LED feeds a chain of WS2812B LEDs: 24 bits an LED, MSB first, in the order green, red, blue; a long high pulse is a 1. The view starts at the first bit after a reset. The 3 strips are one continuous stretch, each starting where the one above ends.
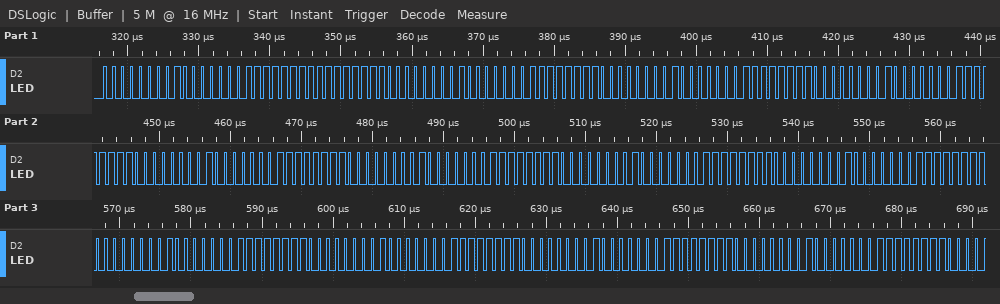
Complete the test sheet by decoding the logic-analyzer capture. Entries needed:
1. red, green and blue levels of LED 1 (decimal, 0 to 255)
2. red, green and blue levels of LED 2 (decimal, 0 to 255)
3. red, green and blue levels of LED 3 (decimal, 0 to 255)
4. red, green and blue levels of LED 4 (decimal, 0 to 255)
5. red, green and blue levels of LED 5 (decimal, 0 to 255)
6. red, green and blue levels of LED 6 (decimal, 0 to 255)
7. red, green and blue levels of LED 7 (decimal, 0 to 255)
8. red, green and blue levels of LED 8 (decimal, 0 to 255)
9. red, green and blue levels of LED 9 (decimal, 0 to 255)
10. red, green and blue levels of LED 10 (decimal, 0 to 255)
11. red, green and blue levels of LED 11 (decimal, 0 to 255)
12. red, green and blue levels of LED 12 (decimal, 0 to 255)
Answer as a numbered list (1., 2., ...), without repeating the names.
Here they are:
1. 128, 0, 255
2. 0, 255, 128
3. 0, 255, 128
4. 0, 255, 128
5. 0, 255, 128
6. 0, 255, 128
7. 0, 255, 128
8. 0, 255, 128
9. 0, 255, 128
10. 0, 255, 128
11. 0, 255, 128
12. 0, 255, 128
